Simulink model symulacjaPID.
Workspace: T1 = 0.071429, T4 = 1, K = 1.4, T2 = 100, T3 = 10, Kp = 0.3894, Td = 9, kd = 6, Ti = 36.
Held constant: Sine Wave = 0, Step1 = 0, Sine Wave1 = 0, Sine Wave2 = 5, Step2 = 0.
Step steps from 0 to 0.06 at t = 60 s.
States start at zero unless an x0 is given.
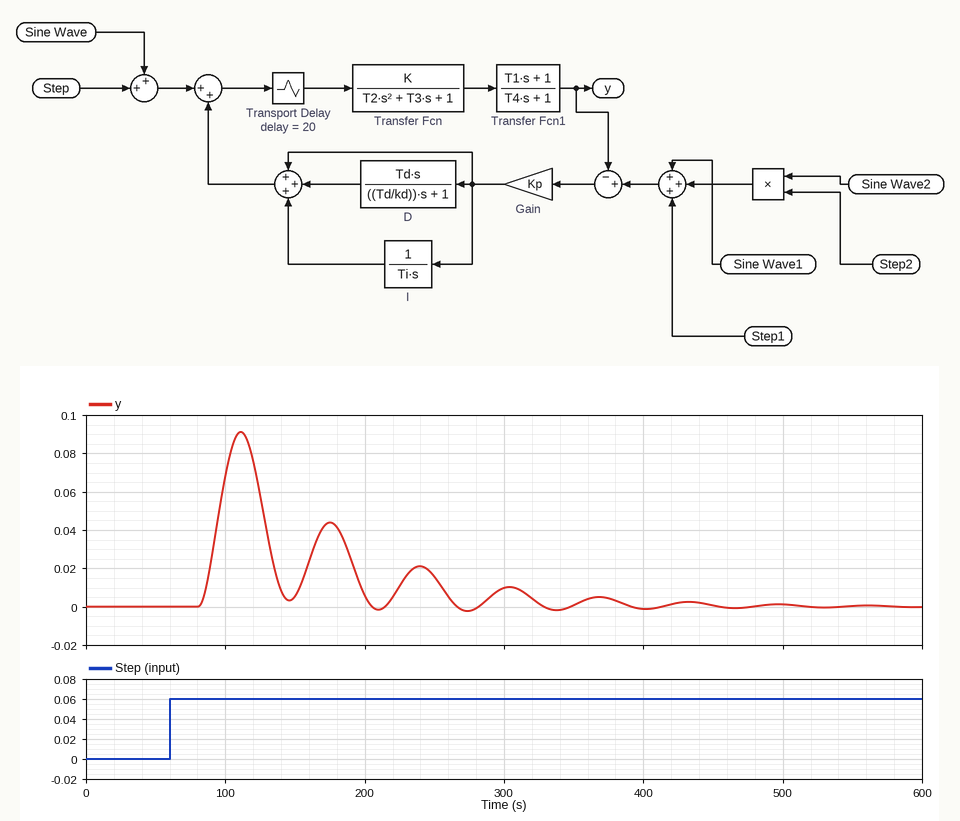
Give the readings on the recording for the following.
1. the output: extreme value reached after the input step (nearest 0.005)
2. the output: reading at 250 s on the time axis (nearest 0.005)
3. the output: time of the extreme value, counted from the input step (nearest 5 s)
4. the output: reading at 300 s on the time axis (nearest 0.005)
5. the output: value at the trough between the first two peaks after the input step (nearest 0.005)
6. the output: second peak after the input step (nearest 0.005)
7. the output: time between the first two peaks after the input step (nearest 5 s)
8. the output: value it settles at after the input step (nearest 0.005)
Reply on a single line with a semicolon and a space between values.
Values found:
0.090; 0.015; 50 s; 0.010; 0.005; 0.045; 65 s; 0.000
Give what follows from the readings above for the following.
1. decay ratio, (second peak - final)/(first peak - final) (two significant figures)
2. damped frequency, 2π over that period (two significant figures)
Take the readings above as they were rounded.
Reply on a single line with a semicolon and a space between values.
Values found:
0.50; 0.097 rad/s
